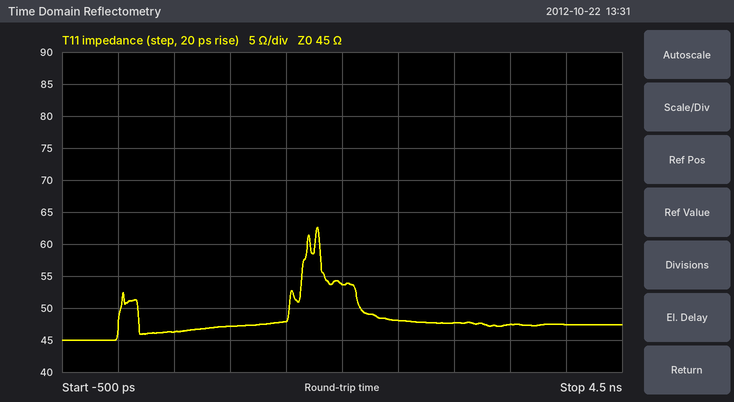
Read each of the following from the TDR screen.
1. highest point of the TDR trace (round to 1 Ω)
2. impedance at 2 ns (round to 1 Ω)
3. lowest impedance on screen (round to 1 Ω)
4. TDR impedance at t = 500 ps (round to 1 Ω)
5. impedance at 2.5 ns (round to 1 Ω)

63 Ω
54 Ω
45 Ω
46 Ω
48 Ω
